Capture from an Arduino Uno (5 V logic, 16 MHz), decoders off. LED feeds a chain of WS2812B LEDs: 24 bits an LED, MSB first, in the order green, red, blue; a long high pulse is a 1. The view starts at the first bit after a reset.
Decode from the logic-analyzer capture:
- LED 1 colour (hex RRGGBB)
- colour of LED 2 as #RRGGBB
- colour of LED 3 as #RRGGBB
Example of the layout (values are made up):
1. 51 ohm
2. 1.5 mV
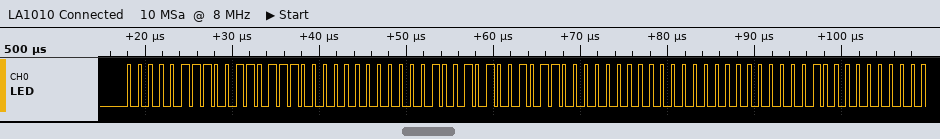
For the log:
1. #370700
2. #4B0900
3. #010000
